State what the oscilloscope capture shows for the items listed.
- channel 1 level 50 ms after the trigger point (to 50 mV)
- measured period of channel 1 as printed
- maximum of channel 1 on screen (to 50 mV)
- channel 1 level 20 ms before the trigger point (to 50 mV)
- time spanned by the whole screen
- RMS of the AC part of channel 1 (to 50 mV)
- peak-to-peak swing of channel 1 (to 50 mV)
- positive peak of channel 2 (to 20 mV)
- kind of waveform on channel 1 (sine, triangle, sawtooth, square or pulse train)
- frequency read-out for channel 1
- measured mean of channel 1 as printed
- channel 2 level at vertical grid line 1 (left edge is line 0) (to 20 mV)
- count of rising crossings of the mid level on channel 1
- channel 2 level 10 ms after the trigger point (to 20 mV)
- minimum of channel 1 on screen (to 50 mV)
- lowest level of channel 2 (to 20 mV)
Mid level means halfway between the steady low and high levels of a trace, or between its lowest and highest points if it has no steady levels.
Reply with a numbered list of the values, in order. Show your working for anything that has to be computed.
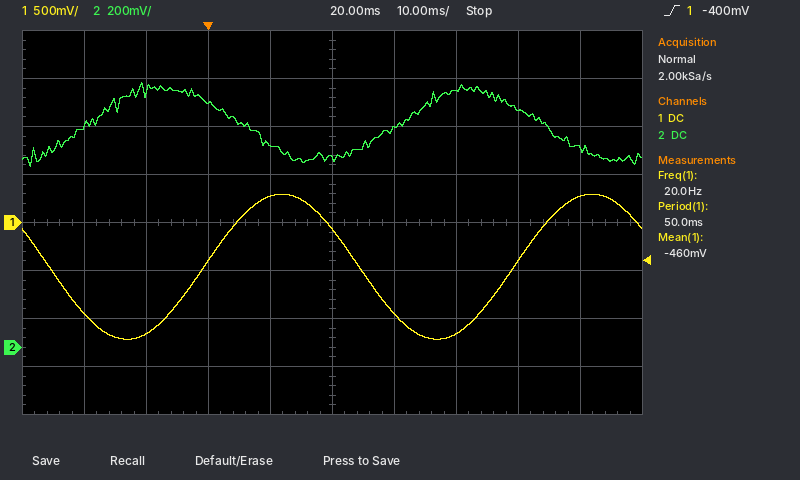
1. -400 mV
2. 50.0 ms
3. 300 mV
4. -950 mV
5. 100 ms
6. 1.50 V / (2√2) ≈ 530 mV, so 550 mV to the nearest 50 mV
7. 300 mV − (-1.20 V) = 1.50 V
8. 1.10 V
9. sine
10. 20.0 Hz
11. -460 mV
12. 920 mV
13. 2
14. 840 mV
15. -1.20 V
16. 760 mV
